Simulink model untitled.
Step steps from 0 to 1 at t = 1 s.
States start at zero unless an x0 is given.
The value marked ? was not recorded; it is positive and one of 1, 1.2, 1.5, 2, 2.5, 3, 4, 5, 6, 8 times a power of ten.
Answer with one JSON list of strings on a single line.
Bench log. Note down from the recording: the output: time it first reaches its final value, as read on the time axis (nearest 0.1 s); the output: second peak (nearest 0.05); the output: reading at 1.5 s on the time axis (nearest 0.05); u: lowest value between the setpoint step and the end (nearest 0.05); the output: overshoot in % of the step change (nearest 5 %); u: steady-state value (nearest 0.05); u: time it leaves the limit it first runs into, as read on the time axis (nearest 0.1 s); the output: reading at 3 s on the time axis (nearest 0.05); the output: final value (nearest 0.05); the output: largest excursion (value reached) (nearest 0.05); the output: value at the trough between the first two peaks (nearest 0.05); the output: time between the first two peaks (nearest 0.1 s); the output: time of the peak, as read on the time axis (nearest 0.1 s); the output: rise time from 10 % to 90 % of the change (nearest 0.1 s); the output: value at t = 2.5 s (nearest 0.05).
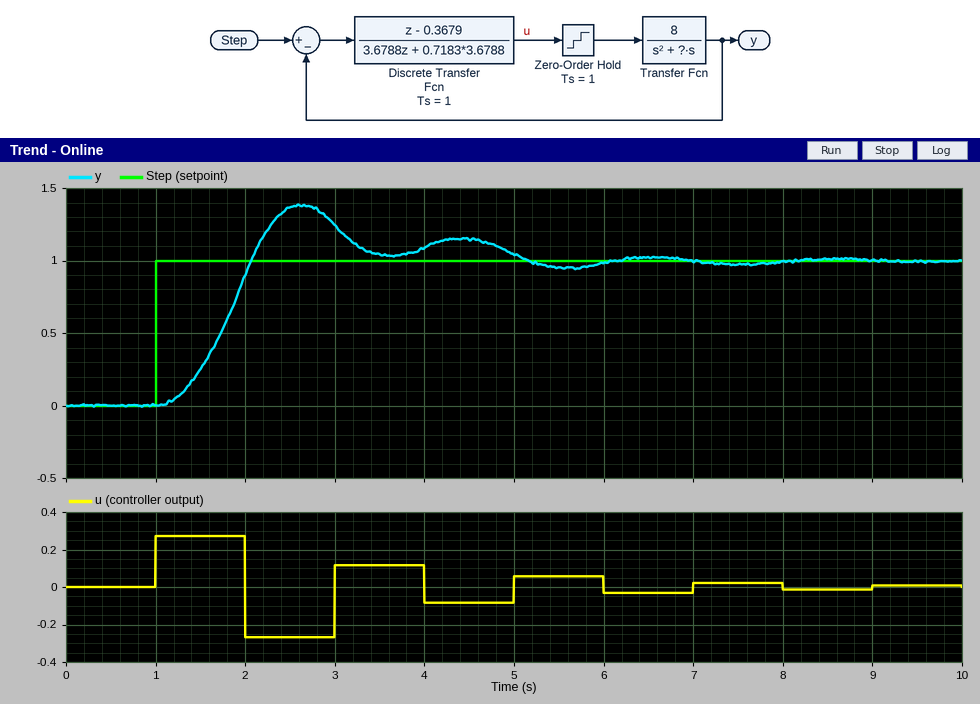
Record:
["2.1 s", "1.15", "0.25", "-0.25", "40 %", "0.00", "2.0 s", "1.25", "1.00", "1.40", "1.05", "1.8 s", "2.6 s", "0.7 s", "1.35"]
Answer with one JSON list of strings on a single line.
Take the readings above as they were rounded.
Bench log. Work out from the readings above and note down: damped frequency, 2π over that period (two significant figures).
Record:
["3.5 rad/s"]
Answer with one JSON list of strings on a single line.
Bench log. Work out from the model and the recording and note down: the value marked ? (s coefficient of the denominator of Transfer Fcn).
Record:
["0.6"]
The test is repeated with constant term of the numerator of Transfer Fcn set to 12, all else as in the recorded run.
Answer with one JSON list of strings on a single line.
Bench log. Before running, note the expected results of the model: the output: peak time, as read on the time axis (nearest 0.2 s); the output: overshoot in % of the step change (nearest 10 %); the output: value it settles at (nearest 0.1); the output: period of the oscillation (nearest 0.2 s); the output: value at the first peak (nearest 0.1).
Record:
["2.4 s", "90 %", "1.0", "2.2 s", "1.9"]
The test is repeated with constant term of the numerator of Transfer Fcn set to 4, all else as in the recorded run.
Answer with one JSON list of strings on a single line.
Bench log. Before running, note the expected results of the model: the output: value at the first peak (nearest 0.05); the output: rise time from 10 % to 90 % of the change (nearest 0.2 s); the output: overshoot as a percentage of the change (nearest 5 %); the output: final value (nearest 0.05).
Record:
["1.10", "2.2 s", "10 %", "1.00"]
